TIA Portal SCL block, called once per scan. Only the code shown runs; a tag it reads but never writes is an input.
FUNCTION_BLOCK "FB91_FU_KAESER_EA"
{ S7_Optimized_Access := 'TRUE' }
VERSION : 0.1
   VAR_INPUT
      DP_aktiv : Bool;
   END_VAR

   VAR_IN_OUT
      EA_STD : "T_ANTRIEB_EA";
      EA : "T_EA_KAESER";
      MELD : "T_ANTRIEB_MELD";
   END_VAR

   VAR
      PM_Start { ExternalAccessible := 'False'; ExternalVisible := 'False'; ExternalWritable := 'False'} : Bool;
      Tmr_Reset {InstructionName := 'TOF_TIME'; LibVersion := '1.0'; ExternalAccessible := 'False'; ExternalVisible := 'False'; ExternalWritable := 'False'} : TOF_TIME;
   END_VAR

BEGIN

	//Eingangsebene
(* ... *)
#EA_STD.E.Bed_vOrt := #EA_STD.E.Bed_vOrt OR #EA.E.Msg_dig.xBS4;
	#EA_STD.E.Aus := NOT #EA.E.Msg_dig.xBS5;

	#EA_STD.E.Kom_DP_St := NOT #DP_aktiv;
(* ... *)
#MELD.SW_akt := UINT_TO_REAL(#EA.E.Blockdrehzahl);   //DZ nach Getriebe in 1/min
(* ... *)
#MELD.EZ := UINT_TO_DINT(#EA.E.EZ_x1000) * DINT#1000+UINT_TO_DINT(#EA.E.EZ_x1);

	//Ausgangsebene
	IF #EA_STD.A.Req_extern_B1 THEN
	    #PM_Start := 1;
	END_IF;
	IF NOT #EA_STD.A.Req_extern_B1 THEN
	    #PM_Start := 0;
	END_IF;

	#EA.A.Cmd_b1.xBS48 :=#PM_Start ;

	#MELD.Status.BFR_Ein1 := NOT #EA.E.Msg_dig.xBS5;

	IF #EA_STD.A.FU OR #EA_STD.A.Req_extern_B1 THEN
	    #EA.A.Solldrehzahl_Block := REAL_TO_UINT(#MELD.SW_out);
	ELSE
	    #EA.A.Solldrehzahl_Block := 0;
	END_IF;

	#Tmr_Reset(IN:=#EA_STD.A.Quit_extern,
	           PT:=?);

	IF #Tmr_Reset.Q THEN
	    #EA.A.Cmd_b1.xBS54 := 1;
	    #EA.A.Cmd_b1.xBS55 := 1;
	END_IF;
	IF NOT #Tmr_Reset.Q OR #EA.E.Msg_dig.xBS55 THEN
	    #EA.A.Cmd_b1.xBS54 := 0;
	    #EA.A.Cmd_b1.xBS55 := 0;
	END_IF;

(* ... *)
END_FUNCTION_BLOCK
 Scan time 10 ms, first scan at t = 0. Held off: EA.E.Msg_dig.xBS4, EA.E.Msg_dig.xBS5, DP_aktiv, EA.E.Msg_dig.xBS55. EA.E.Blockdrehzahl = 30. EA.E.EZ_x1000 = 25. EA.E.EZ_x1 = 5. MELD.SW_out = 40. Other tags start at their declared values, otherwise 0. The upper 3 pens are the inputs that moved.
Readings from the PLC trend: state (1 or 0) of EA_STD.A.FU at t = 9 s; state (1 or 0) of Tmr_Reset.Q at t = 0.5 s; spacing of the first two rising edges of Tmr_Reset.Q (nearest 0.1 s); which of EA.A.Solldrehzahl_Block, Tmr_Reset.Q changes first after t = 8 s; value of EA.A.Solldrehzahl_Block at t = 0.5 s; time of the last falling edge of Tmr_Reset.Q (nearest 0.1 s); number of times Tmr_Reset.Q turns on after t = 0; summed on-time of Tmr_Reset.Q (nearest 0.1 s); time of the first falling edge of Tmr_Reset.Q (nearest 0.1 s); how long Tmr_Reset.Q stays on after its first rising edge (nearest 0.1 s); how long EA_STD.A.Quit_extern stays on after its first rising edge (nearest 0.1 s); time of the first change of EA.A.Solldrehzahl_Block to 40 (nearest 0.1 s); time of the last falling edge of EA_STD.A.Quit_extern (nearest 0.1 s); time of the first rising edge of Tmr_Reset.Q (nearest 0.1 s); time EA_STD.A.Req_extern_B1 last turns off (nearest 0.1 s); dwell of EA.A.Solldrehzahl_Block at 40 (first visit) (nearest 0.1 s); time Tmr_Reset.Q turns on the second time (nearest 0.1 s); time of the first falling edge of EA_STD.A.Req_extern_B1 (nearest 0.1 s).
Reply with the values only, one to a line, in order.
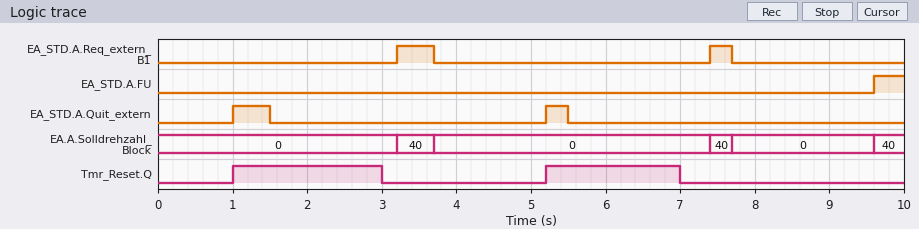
0
0
4.2 s
EA.A.Solldrehzahl_Block
0
7.0 s
2
3.8 s
3.0 s
2.0 s
0.5 s
3.2 s
5.5 s
1.0 s
7.7 s
0.5 s
5.2 s
3.7 s
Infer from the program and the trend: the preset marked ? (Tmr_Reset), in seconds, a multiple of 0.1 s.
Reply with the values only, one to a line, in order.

1.5 s
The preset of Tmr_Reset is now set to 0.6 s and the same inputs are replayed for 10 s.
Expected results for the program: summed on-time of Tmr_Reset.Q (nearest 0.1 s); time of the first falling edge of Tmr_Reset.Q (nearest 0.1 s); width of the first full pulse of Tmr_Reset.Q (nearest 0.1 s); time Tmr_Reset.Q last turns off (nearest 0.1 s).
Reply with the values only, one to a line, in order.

2.0 s
2.1 s
1.1 s
6.1 s
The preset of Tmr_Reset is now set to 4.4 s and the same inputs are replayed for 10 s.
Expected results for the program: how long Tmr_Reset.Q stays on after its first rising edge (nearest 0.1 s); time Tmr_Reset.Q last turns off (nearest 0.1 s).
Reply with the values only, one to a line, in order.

8.9 s
9.9 s
